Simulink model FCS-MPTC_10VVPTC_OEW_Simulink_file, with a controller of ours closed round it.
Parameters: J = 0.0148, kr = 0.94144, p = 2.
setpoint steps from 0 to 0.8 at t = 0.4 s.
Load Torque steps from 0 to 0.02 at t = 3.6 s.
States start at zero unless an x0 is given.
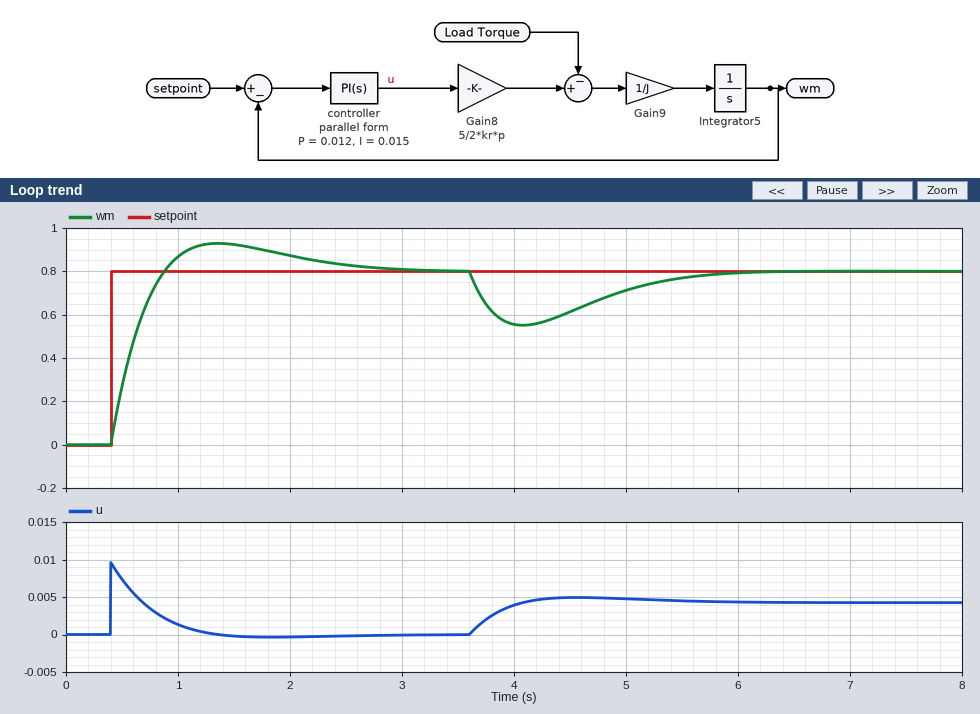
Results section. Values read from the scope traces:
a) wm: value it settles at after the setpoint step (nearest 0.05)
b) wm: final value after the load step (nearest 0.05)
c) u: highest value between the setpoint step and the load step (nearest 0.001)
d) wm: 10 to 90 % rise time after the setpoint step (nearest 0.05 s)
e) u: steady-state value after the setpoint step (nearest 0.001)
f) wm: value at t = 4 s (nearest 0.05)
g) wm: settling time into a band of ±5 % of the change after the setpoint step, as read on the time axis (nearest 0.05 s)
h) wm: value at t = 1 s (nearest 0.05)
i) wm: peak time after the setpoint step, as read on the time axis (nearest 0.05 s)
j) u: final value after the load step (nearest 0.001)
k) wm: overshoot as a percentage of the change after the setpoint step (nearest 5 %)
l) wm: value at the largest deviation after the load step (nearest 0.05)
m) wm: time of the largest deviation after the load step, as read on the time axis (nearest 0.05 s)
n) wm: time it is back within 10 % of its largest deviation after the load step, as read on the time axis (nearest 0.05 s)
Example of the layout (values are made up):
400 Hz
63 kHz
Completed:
0.80
0.80
0.010
0.35 s
0.000
0.55
2.35 s
0.85
1.35 s
0.004
15 %
0.55
4.10 s
5.60 s
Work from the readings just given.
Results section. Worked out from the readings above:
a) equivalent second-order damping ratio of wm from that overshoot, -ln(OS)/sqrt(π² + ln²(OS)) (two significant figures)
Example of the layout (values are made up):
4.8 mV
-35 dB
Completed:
0.52
